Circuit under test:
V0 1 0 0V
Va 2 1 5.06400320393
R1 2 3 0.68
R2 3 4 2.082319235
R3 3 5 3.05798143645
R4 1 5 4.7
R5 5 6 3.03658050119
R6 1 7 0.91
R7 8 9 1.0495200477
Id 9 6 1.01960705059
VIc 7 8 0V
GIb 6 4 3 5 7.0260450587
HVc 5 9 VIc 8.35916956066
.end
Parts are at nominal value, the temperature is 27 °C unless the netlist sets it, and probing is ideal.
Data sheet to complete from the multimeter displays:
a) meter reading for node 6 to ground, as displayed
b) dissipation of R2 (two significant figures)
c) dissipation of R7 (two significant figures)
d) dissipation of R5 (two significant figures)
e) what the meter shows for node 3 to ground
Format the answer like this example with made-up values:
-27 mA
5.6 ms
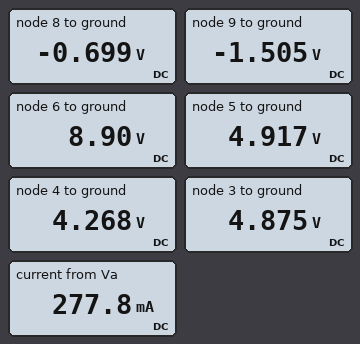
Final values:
8.90 V
180 mW
620 mW
5.2 W
4.875 V
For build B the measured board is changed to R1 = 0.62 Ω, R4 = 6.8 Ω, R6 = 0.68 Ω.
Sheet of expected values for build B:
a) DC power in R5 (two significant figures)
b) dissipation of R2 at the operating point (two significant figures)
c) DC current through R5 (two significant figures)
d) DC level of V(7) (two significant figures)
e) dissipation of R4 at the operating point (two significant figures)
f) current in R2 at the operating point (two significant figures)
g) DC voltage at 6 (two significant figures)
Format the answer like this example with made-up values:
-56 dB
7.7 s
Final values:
3.0 W
840 µW
1.0 A
-520 mV
3.8 W
20 mA
8.1 V
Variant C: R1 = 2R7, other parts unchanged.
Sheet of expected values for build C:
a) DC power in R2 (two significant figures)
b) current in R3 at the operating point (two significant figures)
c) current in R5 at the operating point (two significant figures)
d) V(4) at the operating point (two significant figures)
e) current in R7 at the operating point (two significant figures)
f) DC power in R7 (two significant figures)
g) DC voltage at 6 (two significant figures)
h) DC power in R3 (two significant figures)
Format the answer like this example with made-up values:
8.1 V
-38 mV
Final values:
140 mW
12 mA
1.3 A
3.8 V
690 mA
500 mW
8.3 V
460 µW
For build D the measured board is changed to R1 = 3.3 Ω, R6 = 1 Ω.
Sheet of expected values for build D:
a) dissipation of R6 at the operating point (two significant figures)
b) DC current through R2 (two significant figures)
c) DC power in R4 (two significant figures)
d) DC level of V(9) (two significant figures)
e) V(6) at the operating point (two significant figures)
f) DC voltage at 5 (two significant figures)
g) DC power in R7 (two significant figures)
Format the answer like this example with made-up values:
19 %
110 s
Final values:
470 mW
250 mA
4.0 W
-1.4 V
8.2 V
4.3 V
490 mW
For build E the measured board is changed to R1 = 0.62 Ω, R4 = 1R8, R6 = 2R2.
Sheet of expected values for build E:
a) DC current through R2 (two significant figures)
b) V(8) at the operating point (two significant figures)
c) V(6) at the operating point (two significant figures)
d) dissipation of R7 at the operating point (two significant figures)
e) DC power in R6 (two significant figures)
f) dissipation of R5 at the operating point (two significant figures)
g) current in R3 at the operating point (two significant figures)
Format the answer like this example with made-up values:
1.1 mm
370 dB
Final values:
1.6 A
-1.9 V
12 V
750 mW
1.6 W
21 W
76 mA
